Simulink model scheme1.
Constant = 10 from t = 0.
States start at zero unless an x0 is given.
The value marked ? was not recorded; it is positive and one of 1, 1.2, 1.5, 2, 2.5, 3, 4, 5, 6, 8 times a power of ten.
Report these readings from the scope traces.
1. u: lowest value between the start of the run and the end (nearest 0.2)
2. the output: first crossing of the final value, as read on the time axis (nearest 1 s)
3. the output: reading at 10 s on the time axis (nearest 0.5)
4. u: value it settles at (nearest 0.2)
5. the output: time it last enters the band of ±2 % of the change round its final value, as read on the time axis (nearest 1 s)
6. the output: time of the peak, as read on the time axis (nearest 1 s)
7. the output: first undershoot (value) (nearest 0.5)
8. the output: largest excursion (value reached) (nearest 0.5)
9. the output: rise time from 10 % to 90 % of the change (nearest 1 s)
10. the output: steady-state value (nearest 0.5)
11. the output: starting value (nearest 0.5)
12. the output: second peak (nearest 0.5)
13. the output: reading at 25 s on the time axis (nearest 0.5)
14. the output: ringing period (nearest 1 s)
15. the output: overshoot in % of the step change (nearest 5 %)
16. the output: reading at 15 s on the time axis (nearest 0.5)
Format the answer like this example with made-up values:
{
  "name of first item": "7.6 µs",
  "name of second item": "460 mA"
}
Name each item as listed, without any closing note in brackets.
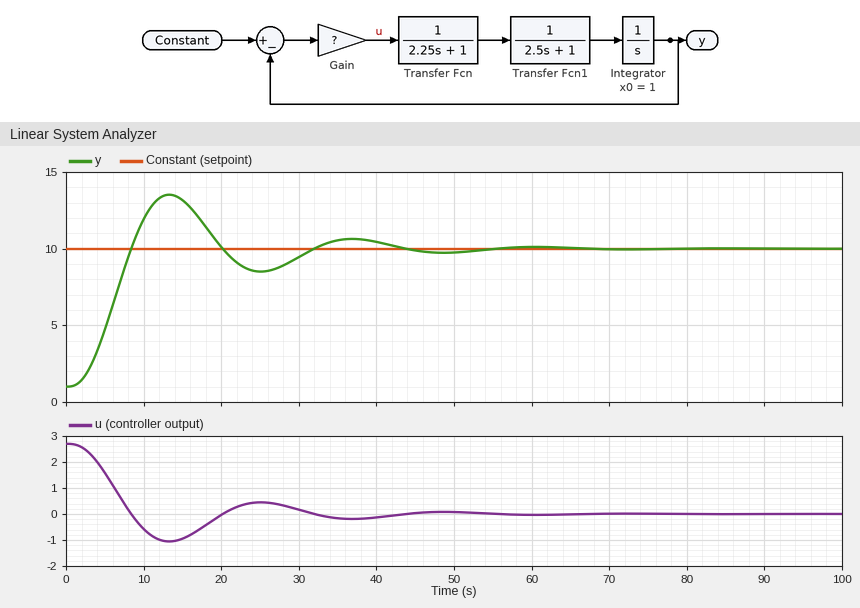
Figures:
{
  "u: lowest value between the start of the run and the end": "-1.0",
  "the output: first crossing of the final value, as read on the time axis": "8 s",
  "the output: reading at 10 s on the time axis": "12.0",
  "u: value it settles at": "0.0",
  "the output: time it last enters the band of ±2 % of the change round its final value, as read on the time axis": "52 s",
  "the output: time of the peak, as read on the time axis": "13 s",
  "the output: first undershoot (value)": "8.5",
  "the output: largest excursion (value reached)": "13.5",
  "the output: rise time from 10 % to 90 % of the change": "5 s",
  "the output: steady-state value": "10.0",
  "the output: starting value": "1.0",
  "the output: second peak": "10.5",
  "the output: reading at 25 s on the time axis": "8.5",
  "the output: ringing period": "24 s",
  "the output: overshoot in % of the step change": "40 %",
  "the output: reading at 15 s on the time axis": "13.0"
}
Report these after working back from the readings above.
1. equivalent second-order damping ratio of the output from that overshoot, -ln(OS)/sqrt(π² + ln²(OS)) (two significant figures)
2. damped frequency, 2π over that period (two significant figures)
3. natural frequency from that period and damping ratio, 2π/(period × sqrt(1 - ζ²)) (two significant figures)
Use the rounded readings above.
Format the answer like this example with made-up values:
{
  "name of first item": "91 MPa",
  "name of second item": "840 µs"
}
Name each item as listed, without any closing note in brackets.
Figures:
{
  "equivalent second-order damping ratio of the output from that overshoot, -ln(OS)/sqrt(π² + ln²(OS))": "0.28",
  "damped frequency, 2π over that period": "0.26 rad/s",
  "natural frequency from that period and damping ratio, 2π/(period × sqrt(1 - ζ²))": "0.27 rad/s"
}
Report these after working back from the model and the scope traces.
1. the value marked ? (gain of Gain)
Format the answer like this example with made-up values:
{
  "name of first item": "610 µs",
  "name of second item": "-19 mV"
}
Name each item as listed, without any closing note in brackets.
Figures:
{
  "the value marked ?": "0.3"
}
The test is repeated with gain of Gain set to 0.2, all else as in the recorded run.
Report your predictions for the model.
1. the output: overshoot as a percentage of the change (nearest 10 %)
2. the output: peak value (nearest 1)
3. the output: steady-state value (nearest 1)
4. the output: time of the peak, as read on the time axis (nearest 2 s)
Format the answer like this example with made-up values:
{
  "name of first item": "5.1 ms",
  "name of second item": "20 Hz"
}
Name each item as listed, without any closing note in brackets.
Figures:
{
  "the output: overshoot as a percentage of the change": "20 %",
  "the output: peak value": "12",
  "the output: steady-state value": "10",
  "the output: time of the peak, as read on the time axis": "16 s"
}
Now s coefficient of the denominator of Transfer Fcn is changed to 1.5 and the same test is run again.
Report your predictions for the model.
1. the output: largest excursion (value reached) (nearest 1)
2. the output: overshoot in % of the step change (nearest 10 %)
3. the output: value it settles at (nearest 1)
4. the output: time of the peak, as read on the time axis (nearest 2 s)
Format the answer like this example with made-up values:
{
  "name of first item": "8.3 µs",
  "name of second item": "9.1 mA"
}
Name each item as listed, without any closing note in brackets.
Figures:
{
  "the output: largest excursion (value reached)": "13",
  "the output: overshoot in % of the step change": "30 %",
  "the output: value it settles at": "10",
  "the output: time of the peak, as read on the time axis": "12 s"
}
